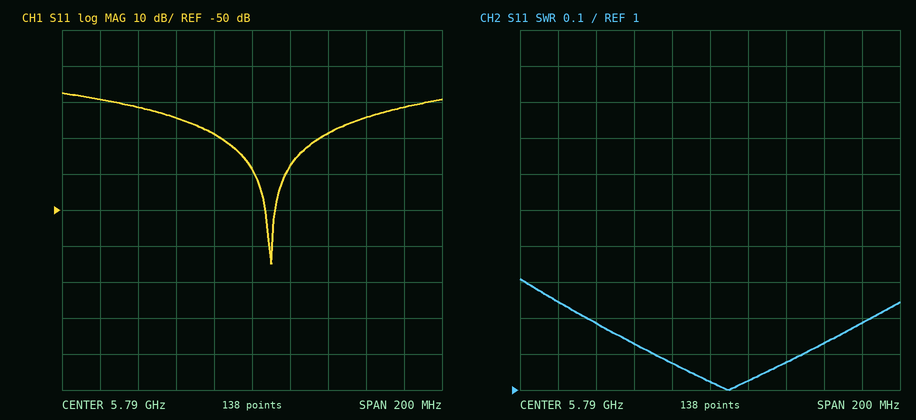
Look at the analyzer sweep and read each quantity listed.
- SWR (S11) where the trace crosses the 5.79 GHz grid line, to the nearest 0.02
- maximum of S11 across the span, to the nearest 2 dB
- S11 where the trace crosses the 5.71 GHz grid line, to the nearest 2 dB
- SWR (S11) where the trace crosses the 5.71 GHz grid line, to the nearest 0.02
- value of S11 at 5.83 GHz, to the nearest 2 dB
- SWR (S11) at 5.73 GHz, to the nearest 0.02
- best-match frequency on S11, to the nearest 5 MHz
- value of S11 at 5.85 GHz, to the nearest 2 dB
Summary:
1.02
-18 dB
-20 dB
1.24
-28 dB
1.18
5.800 GHz
-24 dB
